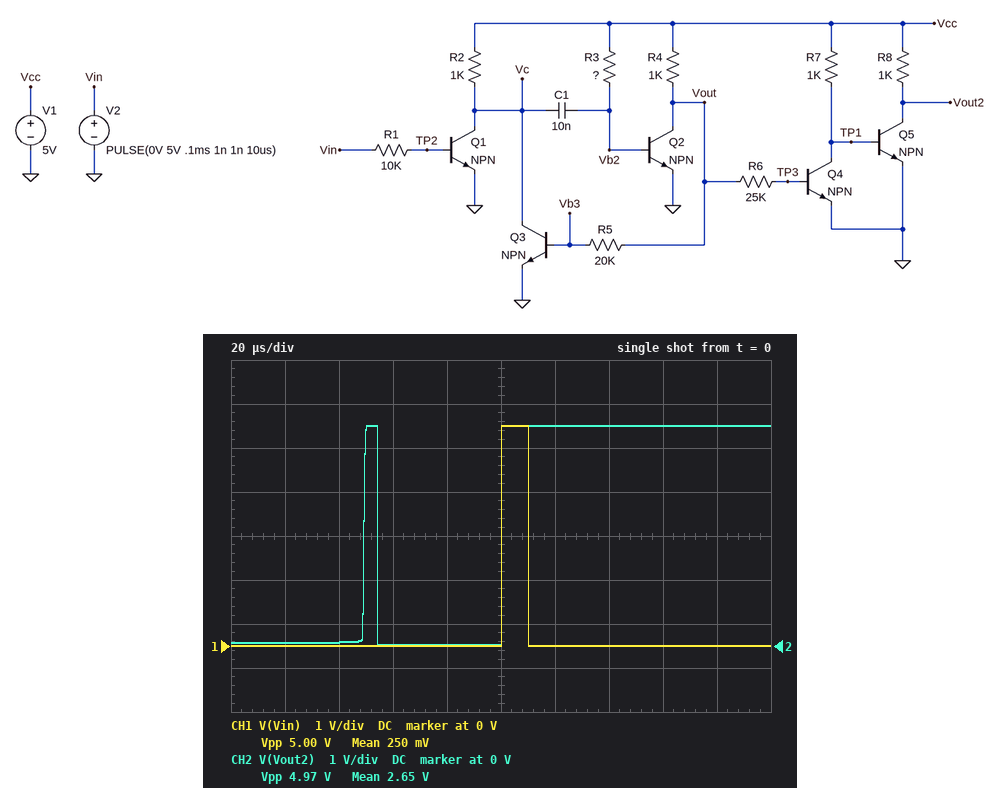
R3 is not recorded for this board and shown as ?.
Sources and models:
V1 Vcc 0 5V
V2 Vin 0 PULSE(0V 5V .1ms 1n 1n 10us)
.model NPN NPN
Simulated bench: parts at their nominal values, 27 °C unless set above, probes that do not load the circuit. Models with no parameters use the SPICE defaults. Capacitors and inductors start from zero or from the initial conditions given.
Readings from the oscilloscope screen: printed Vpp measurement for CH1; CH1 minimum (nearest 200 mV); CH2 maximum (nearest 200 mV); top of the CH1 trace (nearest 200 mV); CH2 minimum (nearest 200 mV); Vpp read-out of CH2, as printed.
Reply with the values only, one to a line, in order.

5.00 V
0 V
5.0 V
5.0 V
0 V
4.97 V
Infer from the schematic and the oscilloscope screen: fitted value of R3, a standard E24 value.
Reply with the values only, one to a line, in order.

27 kΩ
